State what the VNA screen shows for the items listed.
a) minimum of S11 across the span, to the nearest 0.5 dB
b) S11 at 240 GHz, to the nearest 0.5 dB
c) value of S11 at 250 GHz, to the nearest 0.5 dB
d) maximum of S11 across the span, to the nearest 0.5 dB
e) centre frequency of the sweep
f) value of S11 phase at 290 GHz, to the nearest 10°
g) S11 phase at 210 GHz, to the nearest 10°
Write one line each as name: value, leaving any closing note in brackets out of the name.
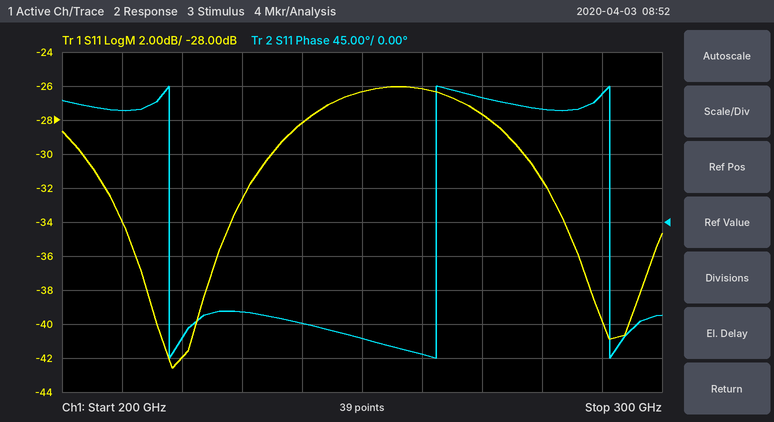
minimum of S11 across the span, to the nearest 0.5 dB: -42.5 dB
S11 at 240 GHz, to the nearest 0.5 dB: -28.0 dB
value of S11 at 250 GHz, to the nearest 0.5 dB: -26.5 dB
maximum of S11 across the span, to the nearest 0.5 dB: -26.0 dB
centre frequency of the sweep: 250 GHz
value of S11 phase at 290 GHz, to the nearest 10°: 170°
S11 phase at 210 GHz, to the nearest 10°: 150°
